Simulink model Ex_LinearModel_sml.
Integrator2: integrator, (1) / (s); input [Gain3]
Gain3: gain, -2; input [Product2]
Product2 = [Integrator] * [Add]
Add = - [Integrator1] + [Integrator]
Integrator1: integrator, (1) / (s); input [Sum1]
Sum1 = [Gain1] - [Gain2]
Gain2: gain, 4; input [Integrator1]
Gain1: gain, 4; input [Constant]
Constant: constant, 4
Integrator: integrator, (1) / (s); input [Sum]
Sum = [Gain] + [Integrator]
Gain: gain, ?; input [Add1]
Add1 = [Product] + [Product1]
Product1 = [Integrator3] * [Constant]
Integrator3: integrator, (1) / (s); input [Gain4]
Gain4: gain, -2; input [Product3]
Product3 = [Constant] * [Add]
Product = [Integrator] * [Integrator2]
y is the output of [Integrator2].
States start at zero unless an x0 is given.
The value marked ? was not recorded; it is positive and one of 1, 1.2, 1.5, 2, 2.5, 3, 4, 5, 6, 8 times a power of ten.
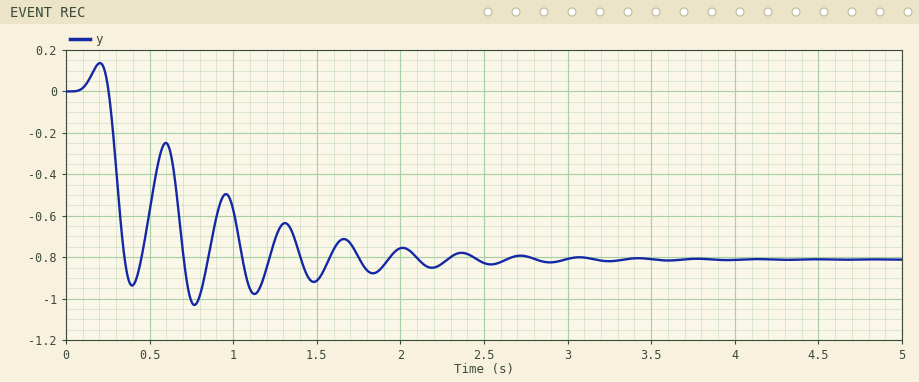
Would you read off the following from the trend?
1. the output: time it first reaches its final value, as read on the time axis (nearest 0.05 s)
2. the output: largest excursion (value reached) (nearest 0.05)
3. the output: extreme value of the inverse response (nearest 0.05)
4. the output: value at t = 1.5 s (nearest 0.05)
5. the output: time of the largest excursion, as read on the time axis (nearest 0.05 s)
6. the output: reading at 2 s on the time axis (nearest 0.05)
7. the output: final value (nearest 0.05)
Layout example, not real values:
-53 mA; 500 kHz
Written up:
0.35 s; -1.05; 0.15; -0.90; 0.75 s; -0.75; -0.80
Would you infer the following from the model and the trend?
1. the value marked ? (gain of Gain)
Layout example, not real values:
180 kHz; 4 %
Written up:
5
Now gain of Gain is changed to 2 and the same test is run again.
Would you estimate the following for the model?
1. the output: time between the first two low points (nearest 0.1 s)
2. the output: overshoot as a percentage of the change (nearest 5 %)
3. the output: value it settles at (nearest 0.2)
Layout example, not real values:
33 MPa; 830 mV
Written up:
0.6 s; 25 %; -1.8
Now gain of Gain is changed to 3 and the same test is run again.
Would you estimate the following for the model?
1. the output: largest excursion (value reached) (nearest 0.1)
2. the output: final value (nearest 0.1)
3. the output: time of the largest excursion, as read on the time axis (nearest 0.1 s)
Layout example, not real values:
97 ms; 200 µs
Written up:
-1.6; -1.3; 1.0 s
